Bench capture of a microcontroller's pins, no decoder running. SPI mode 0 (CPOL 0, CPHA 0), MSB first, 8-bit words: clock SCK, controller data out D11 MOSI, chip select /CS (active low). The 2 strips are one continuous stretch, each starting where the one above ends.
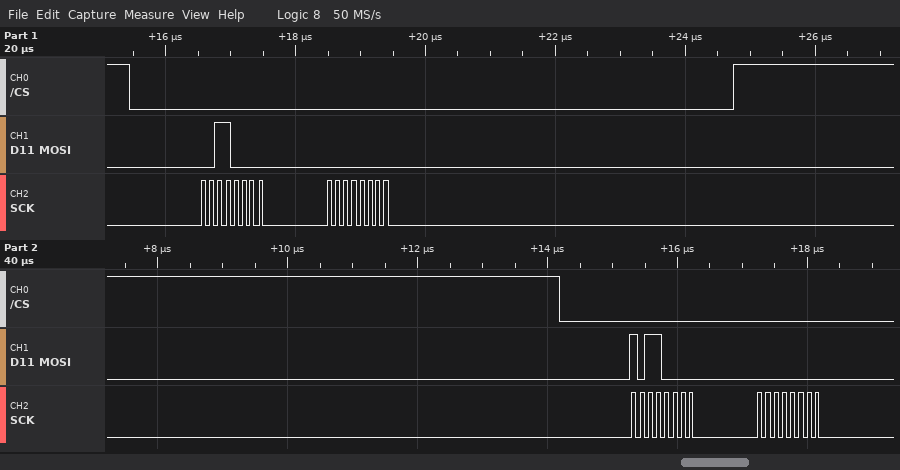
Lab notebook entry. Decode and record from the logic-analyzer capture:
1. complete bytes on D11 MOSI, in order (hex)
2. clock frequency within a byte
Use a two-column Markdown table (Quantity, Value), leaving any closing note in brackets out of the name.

| Quantity | Value |
|---|---|
| complete bytes on D11 MOSI, in order | 30 00 B0 00 |
| clock frequency within a byte | 8 MHz |
